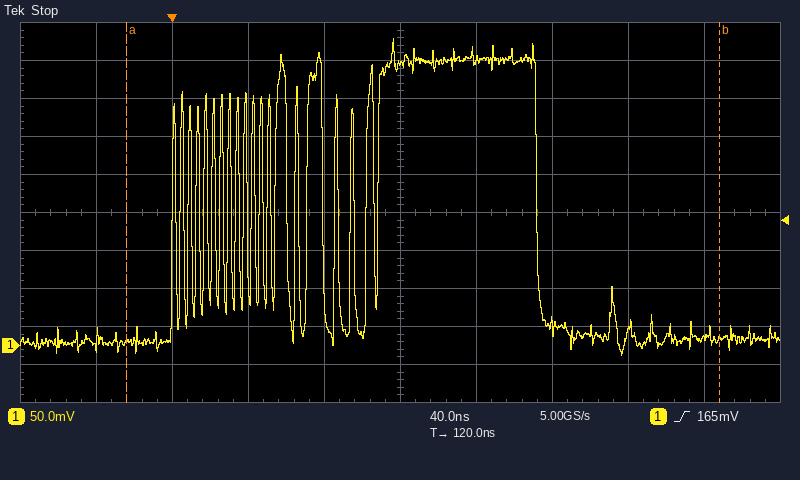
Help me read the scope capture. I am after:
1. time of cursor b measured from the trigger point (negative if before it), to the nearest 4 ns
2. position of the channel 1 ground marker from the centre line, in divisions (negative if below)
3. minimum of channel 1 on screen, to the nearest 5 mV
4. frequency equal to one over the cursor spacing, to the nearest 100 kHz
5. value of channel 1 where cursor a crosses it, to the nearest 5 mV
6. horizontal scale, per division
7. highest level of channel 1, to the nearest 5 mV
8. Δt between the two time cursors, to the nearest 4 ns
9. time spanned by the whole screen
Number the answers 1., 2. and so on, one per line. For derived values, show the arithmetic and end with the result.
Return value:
1. +288 ns
2. -3.5 div
3. -15 mV
4. 1 / 312 ns ≈ 3.2 MHz
5. 5 mV
6. 40 ns
7. 405 mV
8. 312 ns
9. 400 ns
